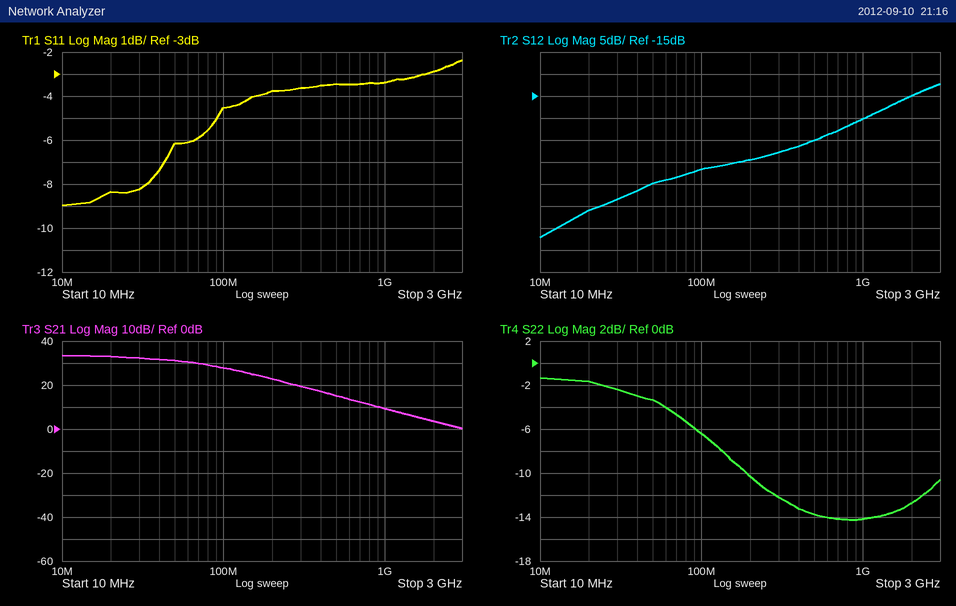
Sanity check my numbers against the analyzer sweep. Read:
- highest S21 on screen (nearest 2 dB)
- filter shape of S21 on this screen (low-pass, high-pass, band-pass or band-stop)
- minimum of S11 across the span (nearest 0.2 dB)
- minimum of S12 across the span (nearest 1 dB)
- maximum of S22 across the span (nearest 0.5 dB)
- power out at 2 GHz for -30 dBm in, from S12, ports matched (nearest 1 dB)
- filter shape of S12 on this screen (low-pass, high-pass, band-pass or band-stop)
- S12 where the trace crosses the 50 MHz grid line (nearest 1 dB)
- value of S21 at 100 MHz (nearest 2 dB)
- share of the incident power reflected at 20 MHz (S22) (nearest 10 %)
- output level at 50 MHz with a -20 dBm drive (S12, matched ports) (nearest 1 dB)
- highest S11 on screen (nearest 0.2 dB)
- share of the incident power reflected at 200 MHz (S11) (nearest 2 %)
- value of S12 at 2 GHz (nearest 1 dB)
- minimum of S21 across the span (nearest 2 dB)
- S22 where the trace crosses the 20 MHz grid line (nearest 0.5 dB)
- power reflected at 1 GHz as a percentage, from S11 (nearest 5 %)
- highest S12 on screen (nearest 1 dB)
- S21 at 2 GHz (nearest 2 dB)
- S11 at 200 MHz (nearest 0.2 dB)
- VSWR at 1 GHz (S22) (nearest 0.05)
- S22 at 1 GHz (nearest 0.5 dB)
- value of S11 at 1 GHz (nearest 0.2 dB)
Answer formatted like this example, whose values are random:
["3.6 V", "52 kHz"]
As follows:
["34 dB", "low-pass", "-9.0 dB", "-47 dB", "-1.5 dB", "-45 dBm", "high-pass", "-35 dB", "28 dB", "70 %", "-55 dBm", "-2.4 dB", "42 %", "-15 dB", "0 dB", "-1.5 dB", "45 %", "-12 dB", "4 dB", "-3.8 dB", "1.50", "-14.0 dB", "-3.4 dB"]
